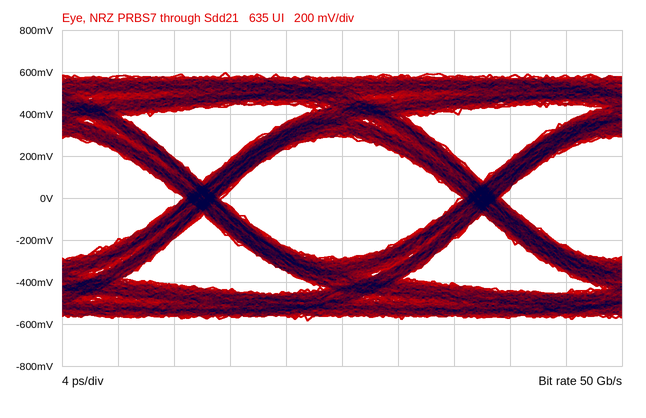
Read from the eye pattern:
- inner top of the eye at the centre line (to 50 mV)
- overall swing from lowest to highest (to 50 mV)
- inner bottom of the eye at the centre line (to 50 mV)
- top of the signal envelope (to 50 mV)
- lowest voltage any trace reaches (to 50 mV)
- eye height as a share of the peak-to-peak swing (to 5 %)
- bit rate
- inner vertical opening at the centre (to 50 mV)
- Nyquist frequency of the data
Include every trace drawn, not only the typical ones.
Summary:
300 mV
1.20 V
-300 mV
600 mV
-600 mV
50 %
50 Gb/s
600 mV
25 GHz
